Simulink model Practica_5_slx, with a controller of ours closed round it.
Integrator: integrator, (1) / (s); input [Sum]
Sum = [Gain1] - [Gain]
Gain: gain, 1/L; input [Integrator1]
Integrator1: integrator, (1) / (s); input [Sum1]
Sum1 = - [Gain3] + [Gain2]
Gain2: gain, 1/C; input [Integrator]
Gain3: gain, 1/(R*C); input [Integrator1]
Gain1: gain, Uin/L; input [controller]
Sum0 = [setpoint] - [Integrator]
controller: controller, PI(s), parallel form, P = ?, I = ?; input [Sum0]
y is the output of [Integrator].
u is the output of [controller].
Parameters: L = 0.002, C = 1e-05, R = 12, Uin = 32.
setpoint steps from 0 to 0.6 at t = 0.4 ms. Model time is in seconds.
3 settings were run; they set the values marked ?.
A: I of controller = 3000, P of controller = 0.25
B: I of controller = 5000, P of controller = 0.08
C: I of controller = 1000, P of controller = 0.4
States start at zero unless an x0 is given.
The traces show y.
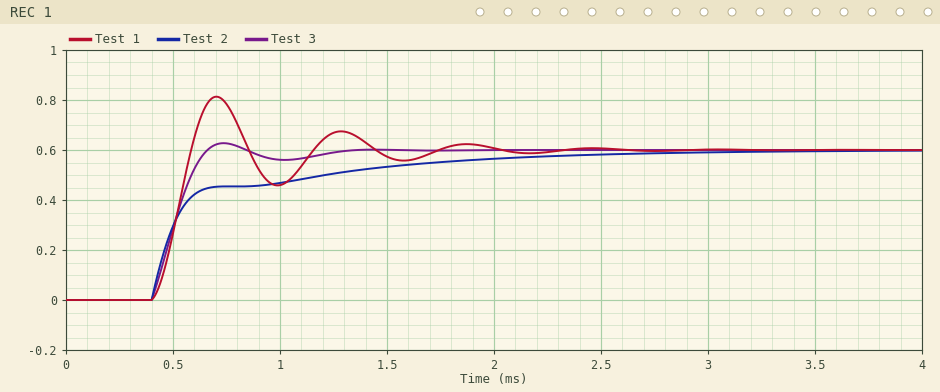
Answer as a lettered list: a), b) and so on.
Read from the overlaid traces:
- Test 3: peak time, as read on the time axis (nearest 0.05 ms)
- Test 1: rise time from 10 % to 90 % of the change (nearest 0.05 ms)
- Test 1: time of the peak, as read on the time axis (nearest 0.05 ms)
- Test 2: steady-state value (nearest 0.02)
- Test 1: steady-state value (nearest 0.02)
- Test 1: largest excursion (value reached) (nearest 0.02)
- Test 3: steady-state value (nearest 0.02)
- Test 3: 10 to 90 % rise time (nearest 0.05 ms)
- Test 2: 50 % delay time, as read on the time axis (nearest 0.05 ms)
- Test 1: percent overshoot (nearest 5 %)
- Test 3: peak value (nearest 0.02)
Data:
a) 0.75 ms
b) 0.15 ms
c) 0.70 ms
d) 0.60
e) 0.60
f) 0.82
g) 0.60
h) 0.20 ms
i) 0.50 ms
j) 35 %
k) 0.62
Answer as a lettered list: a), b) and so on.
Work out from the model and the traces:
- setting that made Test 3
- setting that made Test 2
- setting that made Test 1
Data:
a) A
b) C
c) B
